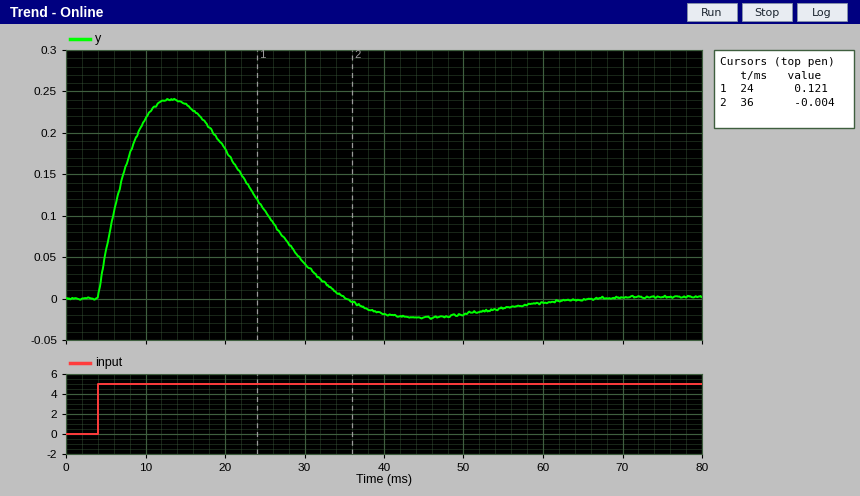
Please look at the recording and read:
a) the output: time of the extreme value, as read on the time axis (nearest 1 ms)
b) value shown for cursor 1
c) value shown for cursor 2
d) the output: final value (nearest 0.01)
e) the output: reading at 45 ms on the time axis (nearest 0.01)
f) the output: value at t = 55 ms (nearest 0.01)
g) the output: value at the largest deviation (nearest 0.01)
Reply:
13 ms
0.121
-0.004
0.00
-0.02
-0.01
0.24
